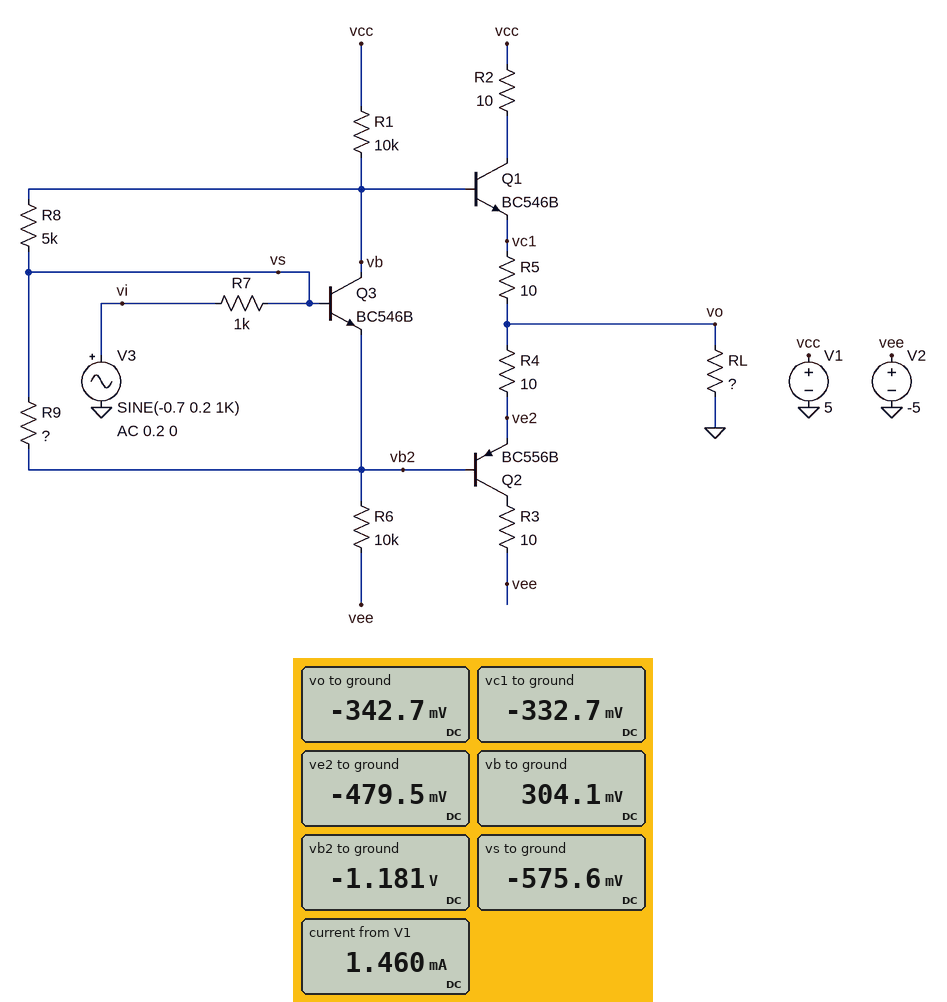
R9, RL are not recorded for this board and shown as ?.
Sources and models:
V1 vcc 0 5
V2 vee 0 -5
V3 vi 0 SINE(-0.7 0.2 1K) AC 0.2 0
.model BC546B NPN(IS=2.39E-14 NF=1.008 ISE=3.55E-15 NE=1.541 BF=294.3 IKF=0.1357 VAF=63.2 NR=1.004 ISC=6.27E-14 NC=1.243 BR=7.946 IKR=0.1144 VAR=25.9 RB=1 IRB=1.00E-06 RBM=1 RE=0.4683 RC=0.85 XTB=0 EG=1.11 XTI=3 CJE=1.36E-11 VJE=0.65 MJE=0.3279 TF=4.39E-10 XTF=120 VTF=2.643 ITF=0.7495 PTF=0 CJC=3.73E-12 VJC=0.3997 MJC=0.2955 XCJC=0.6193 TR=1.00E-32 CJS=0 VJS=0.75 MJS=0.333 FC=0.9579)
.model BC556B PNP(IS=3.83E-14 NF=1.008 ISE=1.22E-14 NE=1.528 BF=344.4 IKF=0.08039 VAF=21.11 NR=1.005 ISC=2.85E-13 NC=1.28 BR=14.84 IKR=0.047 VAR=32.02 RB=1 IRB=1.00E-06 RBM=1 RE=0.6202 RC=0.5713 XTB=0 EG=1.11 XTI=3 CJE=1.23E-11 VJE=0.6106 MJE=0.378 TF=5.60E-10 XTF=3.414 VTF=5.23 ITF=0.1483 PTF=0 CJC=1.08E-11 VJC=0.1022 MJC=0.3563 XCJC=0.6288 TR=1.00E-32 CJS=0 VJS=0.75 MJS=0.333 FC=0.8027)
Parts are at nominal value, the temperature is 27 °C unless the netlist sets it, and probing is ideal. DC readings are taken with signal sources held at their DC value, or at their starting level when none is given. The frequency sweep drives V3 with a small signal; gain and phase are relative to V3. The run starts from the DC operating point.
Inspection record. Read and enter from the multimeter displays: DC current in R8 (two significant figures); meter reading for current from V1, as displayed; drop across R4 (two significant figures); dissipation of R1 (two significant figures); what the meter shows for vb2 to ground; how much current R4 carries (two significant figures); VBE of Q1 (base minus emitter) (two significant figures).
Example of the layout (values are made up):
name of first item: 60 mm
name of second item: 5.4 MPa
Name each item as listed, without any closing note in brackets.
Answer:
DC current in R8: 180 µA
meter reading for current from V1, as displayed: 1.460 mA
drop across R4: 140 mV
dissipation of R1: 2.2 mW
what the meter shows for vb2 to ground: -1.181 V
how much current R4 carries: 14 mA
VBE of Q1 (base minus emitter): 640 mV
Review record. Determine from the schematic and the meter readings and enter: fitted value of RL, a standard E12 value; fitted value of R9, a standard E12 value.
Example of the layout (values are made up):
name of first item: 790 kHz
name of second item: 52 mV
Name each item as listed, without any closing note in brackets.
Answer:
fitted value of RL, a standard E12 value: 27 Ω
fitted value of R9, a standard E12 value: 12 kΩ
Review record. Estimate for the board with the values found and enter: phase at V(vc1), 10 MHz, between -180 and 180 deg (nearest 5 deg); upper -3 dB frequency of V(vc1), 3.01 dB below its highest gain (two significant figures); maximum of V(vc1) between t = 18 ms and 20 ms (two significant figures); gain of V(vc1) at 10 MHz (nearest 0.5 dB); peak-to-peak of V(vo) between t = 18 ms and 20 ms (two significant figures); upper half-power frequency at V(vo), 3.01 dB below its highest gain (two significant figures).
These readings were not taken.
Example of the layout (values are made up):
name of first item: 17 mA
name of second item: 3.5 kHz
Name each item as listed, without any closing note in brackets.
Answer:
phase at V(vc1), 10 MHz, between -180 and 180 deg: -20 deg
upper -3 dB frequency of V(vc1), 3.01 dB below its highest gain: 22 MHz
maximum of V(vc1) between t = 18 ms and 20 ms: -240 mV
gain of V(vc1) at 10 MHz: -8.0 dB
peak-to-peak of V(vo) between t = 18 ms and 20 ms: 190 mV
upper half-power frequency at V(vo), 3.01 dB below its highest gain: 21 MHz
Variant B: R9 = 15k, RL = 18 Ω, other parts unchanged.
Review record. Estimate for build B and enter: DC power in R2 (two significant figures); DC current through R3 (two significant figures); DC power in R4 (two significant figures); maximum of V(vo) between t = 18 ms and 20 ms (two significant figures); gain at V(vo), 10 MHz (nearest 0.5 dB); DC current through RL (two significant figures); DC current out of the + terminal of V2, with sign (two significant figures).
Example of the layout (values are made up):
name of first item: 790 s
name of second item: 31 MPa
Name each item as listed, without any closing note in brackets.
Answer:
DC power in R2: 1.0 µW
DC current through R3: 17 mA
DC power in R4: 2.8 mW
maximum of V(vo) between t = 18 ms and 20 ms: -200 mV
gain at V(vo), 10 MHz: -6.0 dB
DC current through RL: 16 mA
DC current out of the + terminal of V2, with sign: -17 mA
